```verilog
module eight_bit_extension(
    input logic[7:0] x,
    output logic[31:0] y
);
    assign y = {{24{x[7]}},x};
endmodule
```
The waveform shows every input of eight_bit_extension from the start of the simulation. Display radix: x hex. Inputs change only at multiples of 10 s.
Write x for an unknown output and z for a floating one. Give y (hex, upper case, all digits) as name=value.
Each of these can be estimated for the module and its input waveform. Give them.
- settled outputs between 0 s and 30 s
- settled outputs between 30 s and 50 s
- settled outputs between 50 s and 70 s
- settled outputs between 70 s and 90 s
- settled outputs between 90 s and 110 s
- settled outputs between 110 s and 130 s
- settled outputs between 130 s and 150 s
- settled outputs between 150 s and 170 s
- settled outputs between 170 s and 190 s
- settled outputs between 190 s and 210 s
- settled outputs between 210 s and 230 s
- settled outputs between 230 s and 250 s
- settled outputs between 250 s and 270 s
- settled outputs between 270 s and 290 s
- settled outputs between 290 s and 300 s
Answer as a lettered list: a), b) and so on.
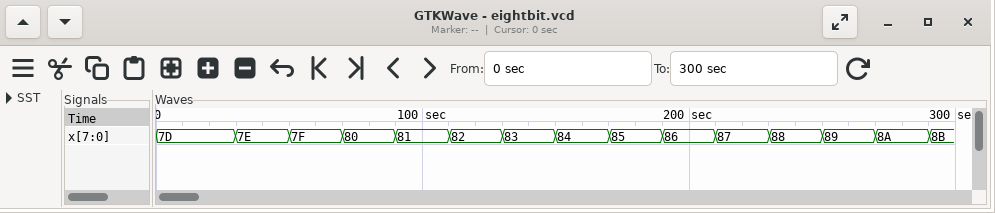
a) y=0000007D
b) y=0000007E
c) y=0000007F
d) y=FFFFFF80
e) y=FFFFFF81
f) y=FFFFFF82
g) y=FFFFFF83
h) y=FFFFFF84
i) y=FFFFFF85
j) y=FFFFFF86
k) y=FFFFFF87
l) y=FFFFFF88
m) y=FFFFFF89
n) y=FFFFFF8A
o) y=FFFFFF8B
